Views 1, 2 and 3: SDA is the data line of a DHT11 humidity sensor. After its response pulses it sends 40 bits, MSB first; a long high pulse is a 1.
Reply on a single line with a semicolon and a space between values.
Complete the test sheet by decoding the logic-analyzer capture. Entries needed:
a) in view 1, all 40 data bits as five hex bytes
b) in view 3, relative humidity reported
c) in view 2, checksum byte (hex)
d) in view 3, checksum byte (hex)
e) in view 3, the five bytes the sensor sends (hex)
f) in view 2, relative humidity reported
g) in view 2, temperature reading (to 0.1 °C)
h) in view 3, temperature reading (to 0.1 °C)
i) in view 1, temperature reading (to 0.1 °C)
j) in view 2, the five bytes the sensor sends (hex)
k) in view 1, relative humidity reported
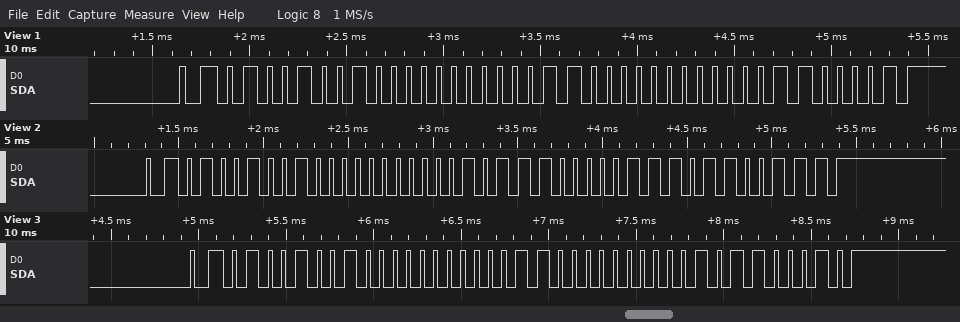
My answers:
49 00 18 00 61; 73 %; 0x67; 0x62; 49 00 18 01 62; 73 %; 23.7 °C; 24.1 °C; 24.0 °C; 49 00 17 07 67; 73 %
